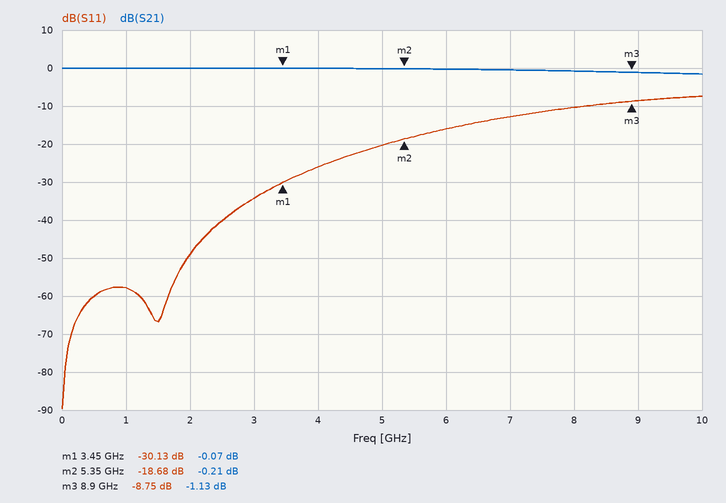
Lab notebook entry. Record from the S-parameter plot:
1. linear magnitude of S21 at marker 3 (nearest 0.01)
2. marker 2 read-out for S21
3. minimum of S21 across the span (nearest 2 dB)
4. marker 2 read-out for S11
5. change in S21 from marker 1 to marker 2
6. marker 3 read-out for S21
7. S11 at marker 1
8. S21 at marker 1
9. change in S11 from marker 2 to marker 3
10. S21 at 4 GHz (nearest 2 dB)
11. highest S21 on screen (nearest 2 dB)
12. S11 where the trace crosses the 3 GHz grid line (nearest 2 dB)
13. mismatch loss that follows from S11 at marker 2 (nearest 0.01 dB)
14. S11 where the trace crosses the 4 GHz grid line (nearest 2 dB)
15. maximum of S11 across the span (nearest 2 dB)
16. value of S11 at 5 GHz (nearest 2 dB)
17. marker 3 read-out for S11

0.88
-0.21 dB
-2 dB
-18.68 dB
-0.14 dB
-1.13 dB
-30.13 dB
-0.07 dB
9.93 dB
0 dB
0 dB
-34 dB
0.06 dB
-26 dB
-8 dB
-20 dB
-8.75 dB
